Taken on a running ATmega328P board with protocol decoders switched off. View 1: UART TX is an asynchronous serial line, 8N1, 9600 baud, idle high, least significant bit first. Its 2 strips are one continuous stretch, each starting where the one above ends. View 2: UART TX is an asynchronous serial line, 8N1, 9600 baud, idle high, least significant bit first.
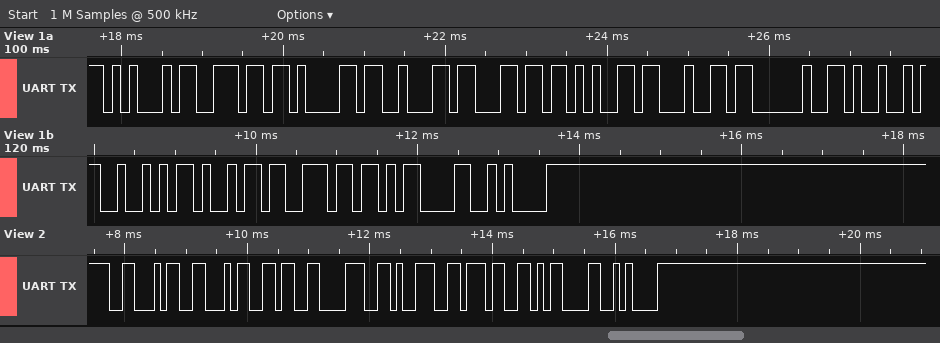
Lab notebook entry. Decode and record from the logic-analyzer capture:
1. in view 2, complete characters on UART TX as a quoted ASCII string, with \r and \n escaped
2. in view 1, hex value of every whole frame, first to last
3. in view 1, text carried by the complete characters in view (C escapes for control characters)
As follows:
"FF6897\r\n"
0x45 0x6E 0x61 0x62 0x6C 0x65 0x64 0x20 0x49 0x52 0x69 0x6E 0x0D 0x0A
"Enabled IRin\r\n"
